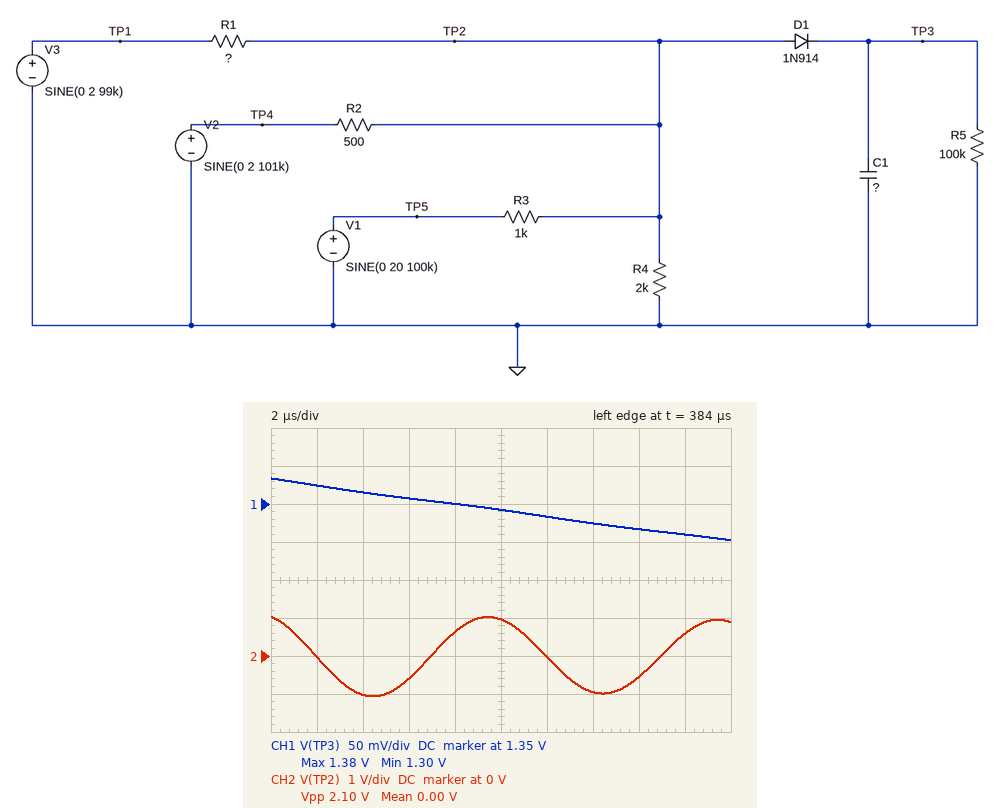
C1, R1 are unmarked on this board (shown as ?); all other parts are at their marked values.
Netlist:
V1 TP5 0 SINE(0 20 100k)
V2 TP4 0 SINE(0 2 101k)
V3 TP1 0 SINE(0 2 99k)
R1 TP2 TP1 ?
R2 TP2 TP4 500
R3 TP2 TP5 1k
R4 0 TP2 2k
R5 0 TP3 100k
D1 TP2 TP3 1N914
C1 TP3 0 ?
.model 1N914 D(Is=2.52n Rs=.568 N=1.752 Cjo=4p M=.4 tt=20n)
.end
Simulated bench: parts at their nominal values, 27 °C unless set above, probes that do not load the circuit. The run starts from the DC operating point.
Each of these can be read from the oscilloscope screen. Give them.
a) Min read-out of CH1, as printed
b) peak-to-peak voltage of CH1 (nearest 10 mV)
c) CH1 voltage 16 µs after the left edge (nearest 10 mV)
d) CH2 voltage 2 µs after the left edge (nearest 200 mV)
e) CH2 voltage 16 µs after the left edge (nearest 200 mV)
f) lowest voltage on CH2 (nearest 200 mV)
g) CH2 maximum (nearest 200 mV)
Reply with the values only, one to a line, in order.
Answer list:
1.30 V
80 mV
1.32 V
0 V
-600 mV
-1.0 V
1.0 V
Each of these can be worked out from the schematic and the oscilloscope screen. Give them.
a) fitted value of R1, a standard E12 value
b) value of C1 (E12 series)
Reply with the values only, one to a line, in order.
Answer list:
180 Ω
3.3 nF
